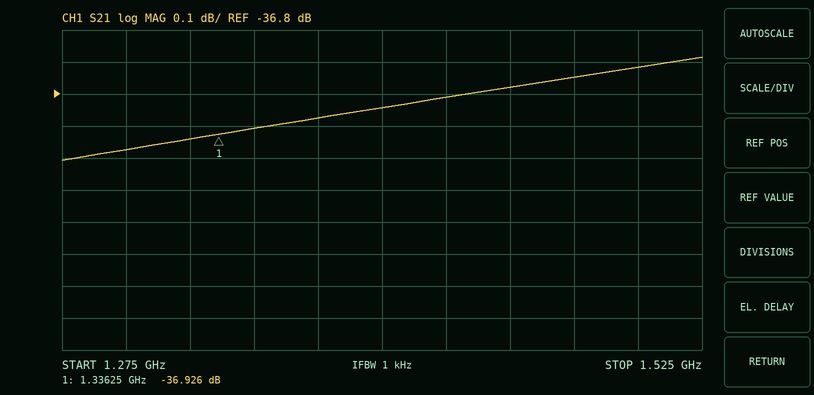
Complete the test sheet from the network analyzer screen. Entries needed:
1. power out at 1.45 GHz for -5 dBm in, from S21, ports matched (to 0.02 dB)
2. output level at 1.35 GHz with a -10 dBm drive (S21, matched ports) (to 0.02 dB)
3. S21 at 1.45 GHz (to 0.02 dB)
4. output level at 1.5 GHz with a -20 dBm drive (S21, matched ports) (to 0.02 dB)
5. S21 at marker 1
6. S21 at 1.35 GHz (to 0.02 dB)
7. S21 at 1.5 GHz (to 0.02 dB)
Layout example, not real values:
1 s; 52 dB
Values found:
-41.78 dBm; -46.90 dBm; -36.78 dB; -56.72 dBm; -36.926 dB; -36.90 dB; -36.72 dB
